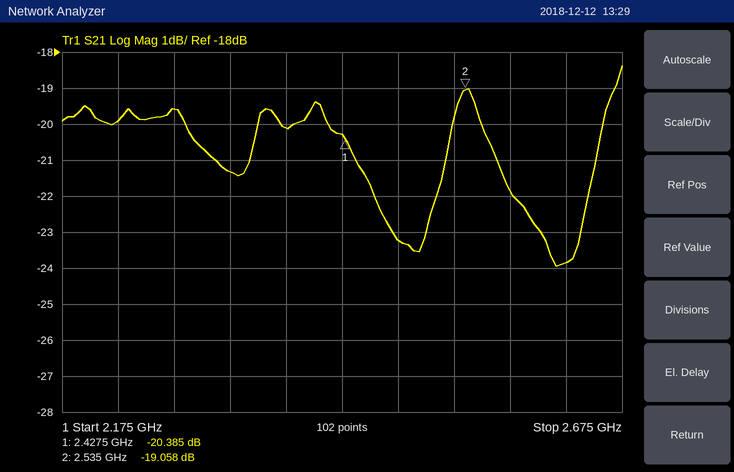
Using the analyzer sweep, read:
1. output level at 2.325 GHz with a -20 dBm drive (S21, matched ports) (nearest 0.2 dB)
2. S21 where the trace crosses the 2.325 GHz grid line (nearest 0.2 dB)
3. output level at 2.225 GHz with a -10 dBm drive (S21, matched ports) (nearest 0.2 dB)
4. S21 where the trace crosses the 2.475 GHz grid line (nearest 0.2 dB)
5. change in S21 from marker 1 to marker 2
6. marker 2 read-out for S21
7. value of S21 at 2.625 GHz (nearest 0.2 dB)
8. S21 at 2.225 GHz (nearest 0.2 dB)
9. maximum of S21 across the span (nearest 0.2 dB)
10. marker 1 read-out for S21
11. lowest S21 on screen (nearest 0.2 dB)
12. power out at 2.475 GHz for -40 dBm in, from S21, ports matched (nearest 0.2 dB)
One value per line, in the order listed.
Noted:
-41.4 dBm
-21.4 dB
-30.0 dBm
-23.2 dB
1.327 dB
-19.058 dB
-23.8 dB
-20.0 dB
-18.4 dB
-20.385 dB
-24.0 dB
-63.2 dBm
